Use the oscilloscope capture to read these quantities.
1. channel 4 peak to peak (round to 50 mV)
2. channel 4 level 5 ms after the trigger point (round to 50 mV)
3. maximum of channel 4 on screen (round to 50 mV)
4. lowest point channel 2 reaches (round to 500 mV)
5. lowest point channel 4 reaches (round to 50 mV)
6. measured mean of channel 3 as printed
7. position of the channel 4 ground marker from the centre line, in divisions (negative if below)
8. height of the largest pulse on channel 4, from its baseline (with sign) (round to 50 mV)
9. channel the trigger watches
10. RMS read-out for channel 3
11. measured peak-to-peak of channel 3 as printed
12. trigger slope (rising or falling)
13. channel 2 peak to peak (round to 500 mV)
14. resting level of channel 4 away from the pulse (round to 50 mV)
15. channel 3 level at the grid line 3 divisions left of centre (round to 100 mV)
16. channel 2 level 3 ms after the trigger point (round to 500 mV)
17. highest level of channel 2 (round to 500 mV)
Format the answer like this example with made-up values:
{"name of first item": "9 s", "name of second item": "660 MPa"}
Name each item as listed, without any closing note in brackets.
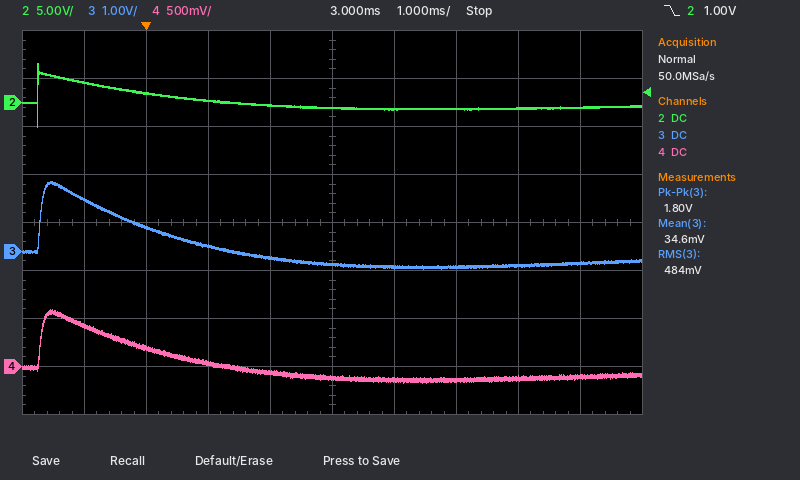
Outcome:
{"channel 4 peak to peak": "750 mV", "channel 4 level 5 ms after the trigger point": "-150 mV", "maximum of channel 4 on screen": "600 mV", "lowest point channel 2 reaches": "-2.5 V", "lowest point channel 4 reaches": "-150 mV", "measured mean of channel 3 as printed": "34.6 mV", "position of the channel 4 ground marker from the centre line, in divisions": "-3.0 div", "height of the largest pulse on channel 4, from its baseline (with sign)": "+700 mV", "channel the trigger watches": "channel 2", "RMS read-out for channel 3": "484 mV", "measured peak-to-peak of channel 3 as printed": "1.80 V", "trigger slope": "falling", "channel 2 peak to peak": "6.5 V", "resting level of channel 4 away from the pulse": "-100 mV", "channel 3 level at the grid line 3 divisions left of centre": "500 mV", "channel 2 level 3 ms after the trigger point": "-500 mV", "highest level of channel 2": "4.0 V"}
